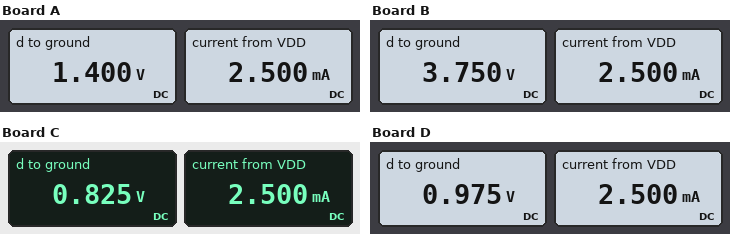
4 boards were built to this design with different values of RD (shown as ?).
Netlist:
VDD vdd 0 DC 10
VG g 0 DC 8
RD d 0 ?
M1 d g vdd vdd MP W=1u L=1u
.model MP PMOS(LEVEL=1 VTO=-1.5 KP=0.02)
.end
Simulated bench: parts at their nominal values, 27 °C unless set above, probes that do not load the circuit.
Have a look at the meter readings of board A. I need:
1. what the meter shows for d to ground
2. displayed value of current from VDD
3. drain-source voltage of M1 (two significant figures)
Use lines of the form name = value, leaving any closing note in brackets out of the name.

what the meter shows for d to ground = 1.400 V
displayed value of current from VDD = 2.500 mA
drain-source voltage of M1 = -8.6 V
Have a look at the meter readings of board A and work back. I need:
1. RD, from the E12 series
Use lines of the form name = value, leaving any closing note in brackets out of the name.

RD, from the E12 series = 560 Ω
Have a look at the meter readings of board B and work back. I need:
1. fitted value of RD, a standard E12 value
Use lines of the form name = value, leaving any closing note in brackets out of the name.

fitted value of RD, a standard E12 value = 1.5 kΩ
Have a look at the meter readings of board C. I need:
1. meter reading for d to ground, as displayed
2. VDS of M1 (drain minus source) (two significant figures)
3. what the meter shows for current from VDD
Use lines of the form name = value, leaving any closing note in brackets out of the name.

meter reading for d to ground, as displayed = 0.825 V
VDS of M1 (drain minus source) = -9.2 V
what the meter shows for current from VDD = 2.500 mA
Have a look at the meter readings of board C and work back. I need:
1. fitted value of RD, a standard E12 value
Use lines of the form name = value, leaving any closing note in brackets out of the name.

fitted value of RD, a standard E12 value = 330 Ω
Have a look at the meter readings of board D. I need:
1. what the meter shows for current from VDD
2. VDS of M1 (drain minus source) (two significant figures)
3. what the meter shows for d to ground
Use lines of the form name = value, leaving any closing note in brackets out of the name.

what the meter shows for current from VDD = 2.500 mA
VDS of M1 (drain minus source) = -9.0 V
what the meter shows for d to ground = 0.975 V
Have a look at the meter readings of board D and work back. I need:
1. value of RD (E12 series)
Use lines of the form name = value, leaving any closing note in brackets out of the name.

value of RD = 390 Ω
